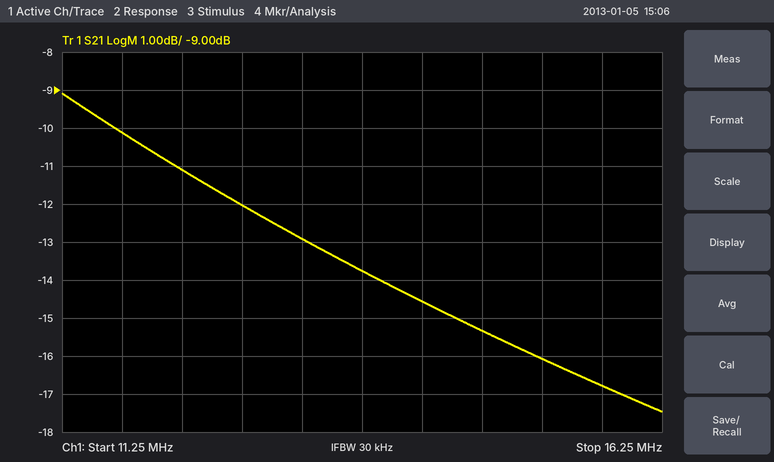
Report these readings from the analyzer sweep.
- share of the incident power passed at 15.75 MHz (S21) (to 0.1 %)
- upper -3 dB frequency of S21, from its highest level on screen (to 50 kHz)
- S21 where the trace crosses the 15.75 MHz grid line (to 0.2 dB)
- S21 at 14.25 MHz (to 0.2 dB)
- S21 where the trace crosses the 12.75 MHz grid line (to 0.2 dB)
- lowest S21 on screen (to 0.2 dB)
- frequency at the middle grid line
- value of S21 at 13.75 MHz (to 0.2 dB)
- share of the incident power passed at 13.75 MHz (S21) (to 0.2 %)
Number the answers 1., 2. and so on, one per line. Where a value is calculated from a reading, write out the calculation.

1. 10^(-16.8/10) ≈ 2.1 %
2. 12.80 MHz
3. -16.8 dB
4. -14.6 dB
5. -12.0 dB
6. -17.4 dB
7. 13.75 MHz
8. -13.8 dB
9. 10^(-13.8/10) ≈ 4.2 %
